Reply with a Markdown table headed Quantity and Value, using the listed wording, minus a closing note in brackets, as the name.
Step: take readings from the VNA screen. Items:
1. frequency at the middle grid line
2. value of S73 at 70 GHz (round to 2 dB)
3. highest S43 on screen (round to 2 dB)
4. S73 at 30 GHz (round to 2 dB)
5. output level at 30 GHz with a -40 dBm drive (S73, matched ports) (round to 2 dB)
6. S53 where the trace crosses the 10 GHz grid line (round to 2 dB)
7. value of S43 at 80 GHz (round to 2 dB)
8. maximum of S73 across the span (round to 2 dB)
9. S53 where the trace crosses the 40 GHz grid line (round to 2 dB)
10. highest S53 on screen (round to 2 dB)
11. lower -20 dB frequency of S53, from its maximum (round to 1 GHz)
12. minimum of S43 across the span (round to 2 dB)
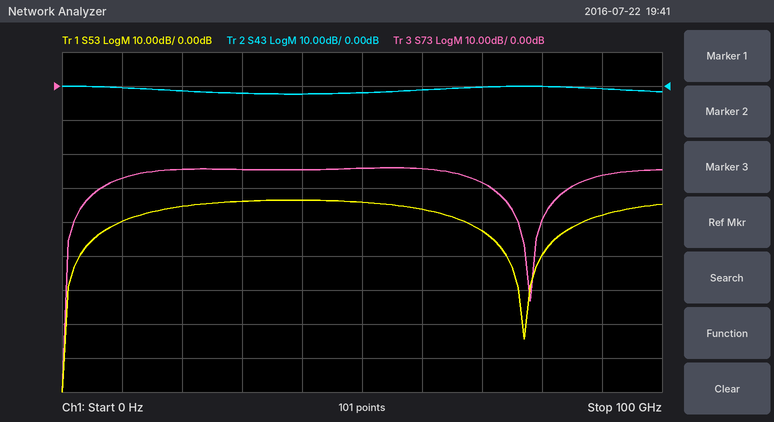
| Quantity | Value |
|---|---|
| frequency at the middle grid line | 50 GHz |
| value of S73 at 70 GHz | -28 dB |
| highest S43 on screen | 0 dB |
| S73 at 30 GHz | -24 dB |
| output level at 30 GHz with a -40 dBm drive (S73, matched ports) | -64 dBm |
| S53 where the trace crosses the 10 GHz grid line | -40 dB |
| value of S43 at 80 GHz | 0 dB |
| maximum of S73 across the span | -24 dB |
| S53 where the trace crosses the 40 GHz grid line | -34 dB |
| highest S53 on screen | -34 dB |
| lower -20 dB frequency of S53, from its maximum | 2 GHz |
| minimum of S43 across the span | -2 dB |
